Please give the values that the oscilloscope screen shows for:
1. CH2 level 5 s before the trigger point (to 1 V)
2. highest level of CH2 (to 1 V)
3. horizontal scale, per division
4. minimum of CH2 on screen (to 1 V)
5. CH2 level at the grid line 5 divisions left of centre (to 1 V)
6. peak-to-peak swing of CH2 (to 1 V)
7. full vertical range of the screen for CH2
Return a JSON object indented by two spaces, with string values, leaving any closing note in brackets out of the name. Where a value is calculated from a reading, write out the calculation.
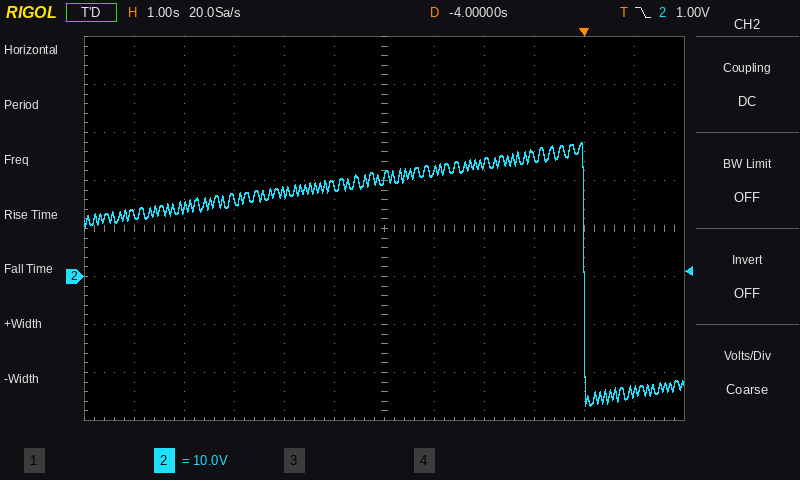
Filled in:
{
  "CH2 level 5 s before the trigger point": "19 V",
  "highest level of CH2": "28 V",
  "horizontal scale, per division": "1 s",
  "minimum of CH2 on screen": "-27 V",
  "CH2 level at the grid line 5 divisions left of centre": "13 V",
  "peak-to-peak swing of CH2": "28 V − (-27 V) = 55 V",
  "full vertical range of the screen for CH2": "80 V"
}
